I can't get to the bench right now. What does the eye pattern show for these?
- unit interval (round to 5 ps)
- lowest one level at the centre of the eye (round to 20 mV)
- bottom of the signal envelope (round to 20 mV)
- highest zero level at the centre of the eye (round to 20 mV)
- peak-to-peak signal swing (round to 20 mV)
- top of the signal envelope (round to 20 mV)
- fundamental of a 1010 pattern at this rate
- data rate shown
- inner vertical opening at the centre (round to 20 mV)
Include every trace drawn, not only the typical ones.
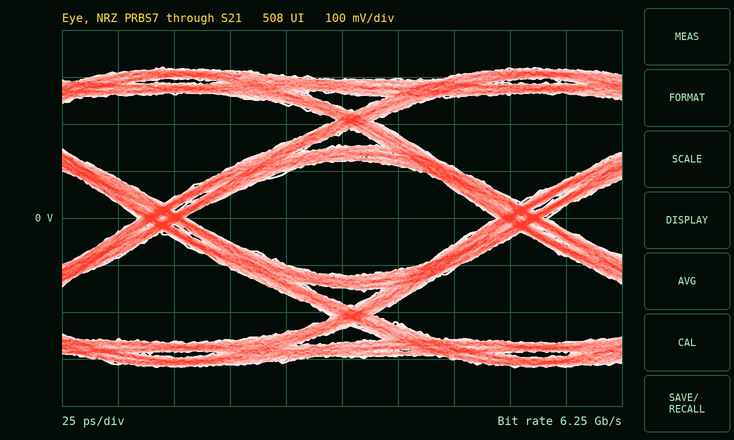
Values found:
160 ps
120 mV
-320 mV
-120 mV
640 mV
320 mV
3.125 GHz
6.25 Gb/s
240 mV
